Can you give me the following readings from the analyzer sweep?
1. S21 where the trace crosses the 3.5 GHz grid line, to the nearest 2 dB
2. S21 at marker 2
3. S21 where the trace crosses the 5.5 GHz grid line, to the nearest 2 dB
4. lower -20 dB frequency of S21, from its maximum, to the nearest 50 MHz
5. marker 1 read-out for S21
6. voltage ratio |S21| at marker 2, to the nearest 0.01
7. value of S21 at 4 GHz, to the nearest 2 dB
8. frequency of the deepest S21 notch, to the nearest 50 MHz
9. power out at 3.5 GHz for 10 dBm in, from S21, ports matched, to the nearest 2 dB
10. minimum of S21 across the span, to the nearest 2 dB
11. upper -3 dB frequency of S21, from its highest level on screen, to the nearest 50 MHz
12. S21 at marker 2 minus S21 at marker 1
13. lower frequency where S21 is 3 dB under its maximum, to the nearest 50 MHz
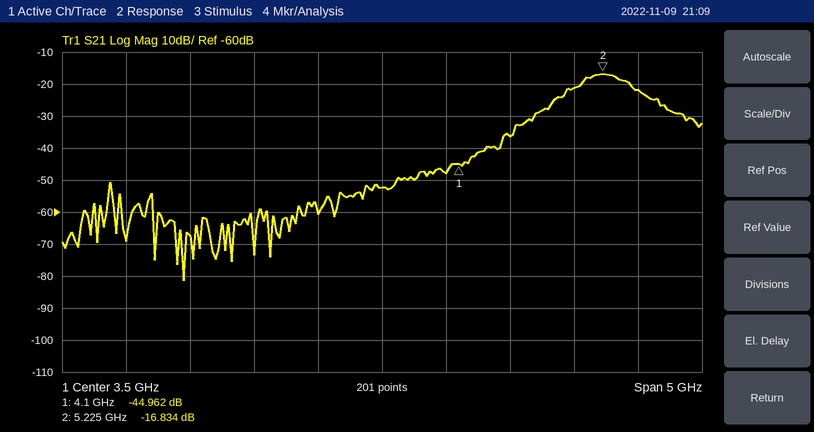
-52 dB
-16.834 dB
-22 dB
4.45 GHz
-44.962 dB
0.14
-48 dB
1.95 GHz
-42 dBm
-82 dB
5.45 GHz
28.128 dB
5.05 GHz
